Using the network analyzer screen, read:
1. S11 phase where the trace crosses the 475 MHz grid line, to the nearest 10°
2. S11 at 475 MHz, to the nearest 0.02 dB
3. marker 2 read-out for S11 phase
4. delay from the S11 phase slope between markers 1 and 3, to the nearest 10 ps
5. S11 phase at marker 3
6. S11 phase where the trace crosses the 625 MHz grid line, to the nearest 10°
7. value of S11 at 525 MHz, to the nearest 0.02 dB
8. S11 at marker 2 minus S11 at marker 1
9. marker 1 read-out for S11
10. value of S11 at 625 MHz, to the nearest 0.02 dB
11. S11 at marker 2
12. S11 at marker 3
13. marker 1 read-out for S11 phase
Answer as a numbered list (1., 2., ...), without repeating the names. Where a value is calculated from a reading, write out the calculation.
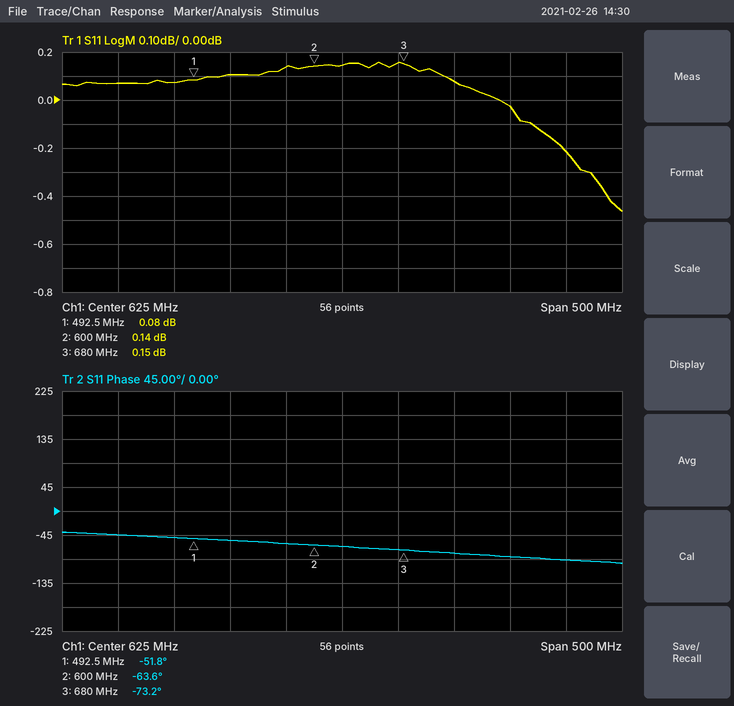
1. -50°
2. 0.08 dB
3. -63.6°
4. −(-73.2° − (-51.8°))/(360° × 187.5 MHz) ≈ 317 ps, so 320 ps to the nearest 10 ps
5. -73.2°
6. -70°
7. 0.10 dB
8. 0.14 − (0.08) = 0.06 dB
9. 0.08 dB
10. 0.14 dB
11. 0.14 dB
12. 0.15 dB
13. -51.8°
